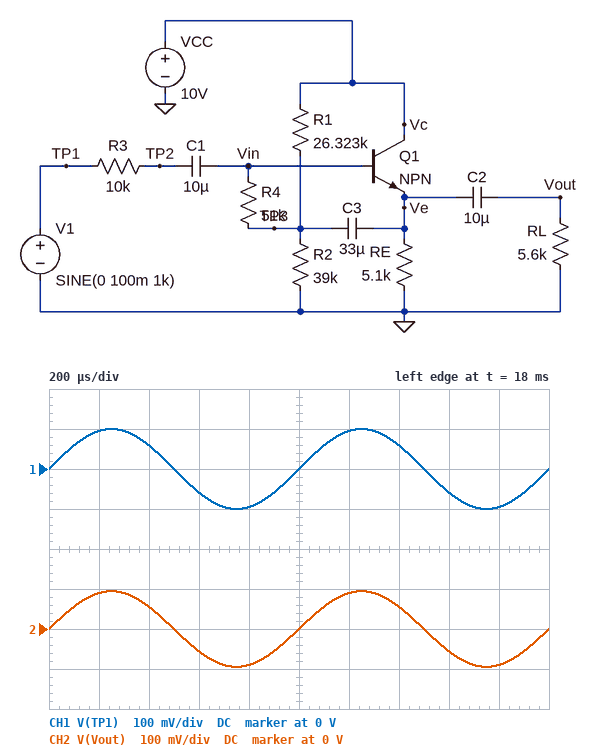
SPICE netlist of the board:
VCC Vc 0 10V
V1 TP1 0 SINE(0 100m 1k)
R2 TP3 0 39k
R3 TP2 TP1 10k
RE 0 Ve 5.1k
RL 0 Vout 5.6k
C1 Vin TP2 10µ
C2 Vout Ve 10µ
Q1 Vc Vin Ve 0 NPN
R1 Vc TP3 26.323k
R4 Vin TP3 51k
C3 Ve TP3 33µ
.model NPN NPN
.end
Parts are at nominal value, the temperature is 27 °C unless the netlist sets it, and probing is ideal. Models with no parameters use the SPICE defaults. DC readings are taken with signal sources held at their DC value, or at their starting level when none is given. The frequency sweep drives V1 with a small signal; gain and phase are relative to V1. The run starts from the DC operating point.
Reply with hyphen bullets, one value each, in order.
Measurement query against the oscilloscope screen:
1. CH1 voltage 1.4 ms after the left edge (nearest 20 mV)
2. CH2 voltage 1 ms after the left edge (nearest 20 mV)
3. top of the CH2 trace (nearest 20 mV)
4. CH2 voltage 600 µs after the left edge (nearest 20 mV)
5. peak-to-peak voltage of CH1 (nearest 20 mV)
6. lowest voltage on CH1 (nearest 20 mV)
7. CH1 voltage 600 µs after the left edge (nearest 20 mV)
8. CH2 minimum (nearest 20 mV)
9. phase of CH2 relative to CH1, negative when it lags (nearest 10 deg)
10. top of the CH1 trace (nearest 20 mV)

- 60 mV
- 0 V
- 100 mV
- -60 mV
- 200 mV
- -100 mV
- -60 mV
- -100 mV
- 0 deg
- 100 mV
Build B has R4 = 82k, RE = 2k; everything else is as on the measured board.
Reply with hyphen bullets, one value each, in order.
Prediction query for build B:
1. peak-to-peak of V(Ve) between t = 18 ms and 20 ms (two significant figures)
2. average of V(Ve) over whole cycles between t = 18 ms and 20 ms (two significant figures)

- 180 mV
- 3.5 V
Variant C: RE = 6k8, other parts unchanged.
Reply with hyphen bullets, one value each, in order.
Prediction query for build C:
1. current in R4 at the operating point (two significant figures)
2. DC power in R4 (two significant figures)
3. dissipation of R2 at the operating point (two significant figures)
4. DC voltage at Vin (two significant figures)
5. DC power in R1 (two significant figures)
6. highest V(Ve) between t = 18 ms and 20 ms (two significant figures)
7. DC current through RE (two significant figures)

- 6.9 µA
- 2.4 µW
- 880 µW
- 5.5 V
- 650 µW
- 4.8 V
- 700 µA
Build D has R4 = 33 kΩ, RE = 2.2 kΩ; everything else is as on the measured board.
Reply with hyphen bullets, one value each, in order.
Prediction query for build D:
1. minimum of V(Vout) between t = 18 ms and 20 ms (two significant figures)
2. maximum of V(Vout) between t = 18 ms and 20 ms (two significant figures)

- -93 mV
- 92 mV
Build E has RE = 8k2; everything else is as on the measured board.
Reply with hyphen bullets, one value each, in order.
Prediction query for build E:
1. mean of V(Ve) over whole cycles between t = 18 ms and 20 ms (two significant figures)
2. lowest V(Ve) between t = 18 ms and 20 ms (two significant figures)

- 4.8 V
- 4.7 V
